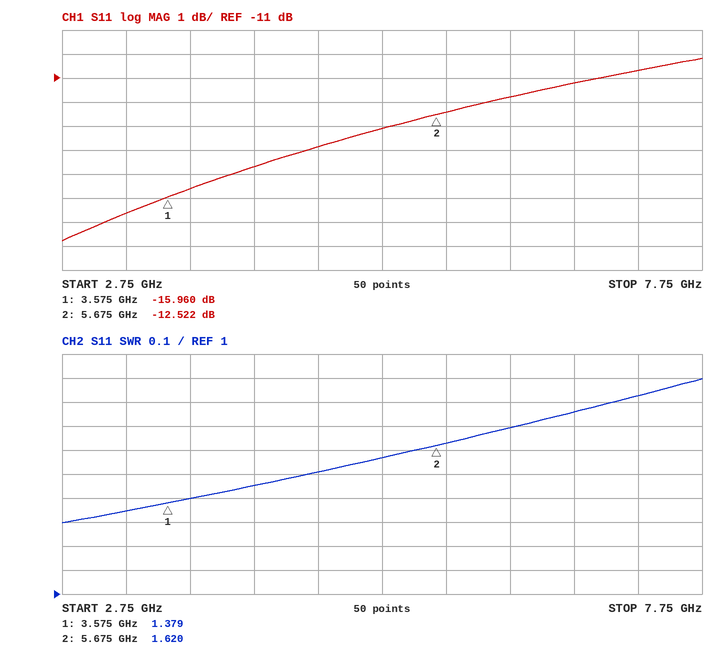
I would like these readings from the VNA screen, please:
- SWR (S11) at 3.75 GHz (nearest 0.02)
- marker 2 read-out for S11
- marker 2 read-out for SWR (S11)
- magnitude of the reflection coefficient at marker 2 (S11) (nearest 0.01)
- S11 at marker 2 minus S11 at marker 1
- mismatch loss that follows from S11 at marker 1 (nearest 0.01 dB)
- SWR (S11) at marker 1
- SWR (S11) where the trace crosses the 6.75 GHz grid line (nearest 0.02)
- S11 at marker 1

1.40
-12.522 dB
1.620
0.24
3.438 dB
0.11 dB
1.379
1.76
-15.960 dB
